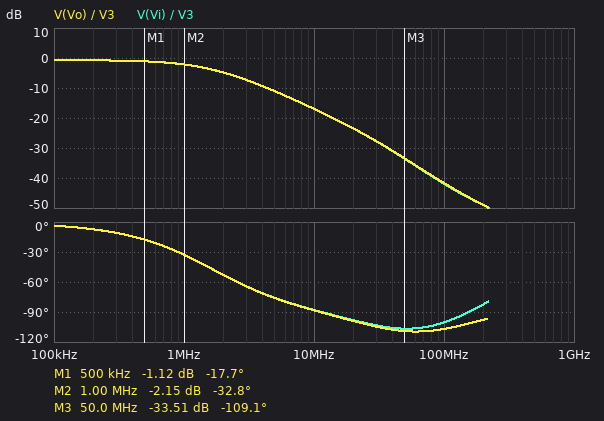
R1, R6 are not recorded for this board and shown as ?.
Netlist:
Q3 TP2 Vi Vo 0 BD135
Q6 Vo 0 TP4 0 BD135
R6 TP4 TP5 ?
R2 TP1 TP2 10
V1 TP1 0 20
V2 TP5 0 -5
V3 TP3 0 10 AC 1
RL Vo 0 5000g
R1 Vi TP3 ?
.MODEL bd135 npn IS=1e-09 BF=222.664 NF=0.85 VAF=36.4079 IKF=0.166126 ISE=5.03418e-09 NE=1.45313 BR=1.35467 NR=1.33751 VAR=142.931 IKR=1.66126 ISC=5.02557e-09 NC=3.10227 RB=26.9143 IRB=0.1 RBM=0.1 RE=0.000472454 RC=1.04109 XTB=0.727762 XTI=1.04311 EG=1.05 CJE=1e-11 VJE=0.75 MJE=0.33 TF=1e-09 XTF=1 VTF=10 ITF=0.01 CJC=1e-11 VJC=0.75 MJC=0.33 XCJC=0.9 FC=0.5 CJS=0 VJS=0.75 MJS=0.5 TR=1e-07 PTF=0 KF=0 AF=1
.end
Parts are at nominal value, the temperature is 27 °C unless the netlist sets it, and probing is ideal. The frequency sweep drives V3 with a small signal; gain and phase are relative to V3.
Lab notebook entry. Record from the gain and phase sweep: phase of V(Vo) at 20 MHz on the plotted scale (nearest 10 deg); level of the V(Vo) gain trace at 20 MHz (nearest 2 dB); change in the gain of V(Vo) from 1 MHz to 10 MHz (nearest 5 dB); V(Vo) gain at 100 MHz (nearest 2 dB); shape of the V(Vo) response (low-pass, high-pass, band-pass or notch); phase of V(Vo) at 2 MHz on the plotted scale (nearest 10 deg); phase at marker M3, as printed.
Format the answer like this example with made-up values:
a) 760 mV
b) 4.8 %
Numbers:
a) -100 deg
b) -24 dB
c) -15 dB
d) -42 dB
e) low-pass
f) -50 deg
g) -109.1 deg
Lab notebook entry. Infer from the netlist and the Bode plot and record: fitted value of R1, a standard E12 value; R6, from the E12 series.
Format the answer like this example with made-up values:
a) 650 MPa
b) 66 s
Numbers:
a) 27 kΩ
b) 180 Ω
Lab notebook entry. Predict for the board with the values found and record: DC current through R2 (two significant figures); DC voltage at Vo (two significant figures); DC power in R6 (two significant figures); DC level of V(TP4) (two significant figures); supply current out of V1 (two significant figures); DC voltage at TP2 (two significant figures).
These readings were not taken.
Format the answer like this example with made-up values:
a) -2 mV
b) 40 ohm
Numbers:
a) 25 mA
b) 4.7 V
c) 120 mW
d) -380 mV
e) 25 mA
f) 20 V
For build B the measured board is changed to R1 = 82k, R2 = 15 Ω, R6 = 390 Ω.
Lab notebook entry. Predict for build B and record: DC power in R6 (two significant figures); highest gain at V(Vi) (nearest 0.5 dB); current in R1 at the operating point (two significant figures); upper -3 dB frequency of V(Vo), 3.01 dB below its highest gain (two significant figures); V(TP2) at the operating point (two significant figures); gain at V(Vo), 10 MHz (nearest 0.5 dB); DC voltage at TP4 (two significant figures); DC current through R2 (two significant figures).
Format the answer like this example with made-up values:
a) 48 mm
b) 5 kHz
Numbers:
a) 55 mW
b) -1.0 dB
c) 93 µA
d) 600 kHz
e) 20 V
f) -25.5 dB
g) -360 mV
h) 12 mA
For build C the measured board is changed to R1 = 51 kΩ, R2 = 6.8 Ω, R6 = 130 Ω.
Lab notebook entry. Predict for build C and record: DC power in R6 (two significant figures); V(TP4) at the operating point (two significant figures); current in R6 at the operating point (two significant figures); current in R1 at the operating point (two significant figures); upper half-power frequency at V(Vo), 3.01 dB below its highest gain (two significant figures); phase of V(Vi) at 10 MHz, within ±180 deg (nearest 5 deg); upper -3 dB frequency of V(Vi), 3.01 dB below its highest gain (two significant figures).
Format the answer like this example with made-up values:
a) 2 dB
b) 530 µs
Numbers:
a) 160 mW
b) -480 mV
c) 35 mA
d) 200 µA
e) 670 kHz
f) -80 deg
g) 680 kHz
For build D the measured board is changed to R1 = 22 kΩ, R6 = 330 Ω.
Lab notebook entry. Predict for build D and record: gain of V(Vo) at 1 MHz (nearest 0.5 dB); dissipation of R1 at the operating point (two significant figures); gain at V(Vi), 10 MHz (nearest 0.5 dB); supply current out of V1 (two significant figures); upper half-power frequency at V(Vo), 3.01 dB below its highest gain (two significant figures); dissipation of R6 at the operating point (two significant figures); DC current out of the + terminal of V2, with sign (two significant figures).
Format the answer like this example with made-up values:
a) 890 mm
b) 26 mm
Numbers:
a) -1.5 dB
b) 290 µW
c) -15.0 dB
d) 14 mA
e) 1.9 MHz
f) 65 mW
g) -14 mA
